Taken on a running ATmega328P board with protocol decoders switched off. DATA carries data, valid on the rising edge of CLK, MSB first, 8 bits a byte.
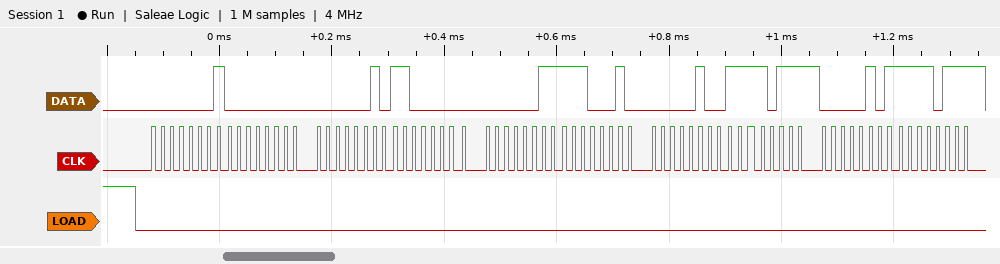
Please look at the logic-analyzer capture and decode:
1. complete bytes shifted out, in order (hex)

01 00 02 C0 03 E2 04 F7 05 F7
